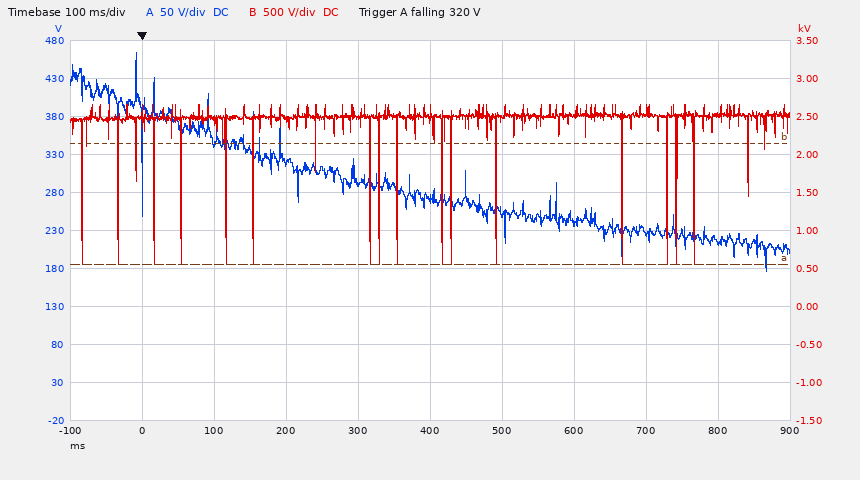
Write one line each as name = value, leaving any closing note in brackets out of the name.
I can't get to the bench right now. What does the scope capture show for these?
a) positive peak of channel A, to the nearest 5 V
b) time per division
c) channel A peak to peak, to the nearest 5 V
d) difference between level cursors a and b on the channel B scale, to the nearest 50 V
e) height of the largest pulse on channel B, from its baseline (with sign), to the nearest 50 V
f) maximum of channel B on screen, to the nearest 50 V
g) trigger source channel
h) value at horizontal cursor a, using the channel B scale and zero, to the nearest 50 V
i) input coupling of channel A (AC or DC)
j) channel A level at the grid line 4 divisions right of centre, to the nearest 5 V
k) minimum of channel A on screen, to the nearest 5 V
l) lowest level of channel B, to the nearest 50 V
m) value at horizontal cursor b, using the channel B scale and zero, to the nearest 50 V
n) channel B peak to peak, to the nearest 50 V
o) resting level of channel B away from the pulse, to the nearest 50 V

positive peak of channel A, to the nearest 5 V = 465 V
time per division = 100 ms
channel A peak to peak, to the nearest 5 V = 290 V
difference between level cursors a and b on the channel B scale, to the nearest 50 V = 1.60 kV
height of the largest pulse on channel B, from its baseline (with sign), to the nearest 50 V = -1.95 kV
maximum of channel B on screen, to the nearest 50 V = 2.65 kV
trigger source channel = channel A
value at horizontal cursor a, using the channel B scale and zero, to the nearest 50 V = 550 V
input coupling of channel A = DC
channel A level at the grid line 4 divisions right of centre, to the nearest 5 V = 215 V
minimum of channel A on screen, to the nearest 5 V = 175 V
lowest level of channel B, to the nearest 50 V = 550 V
value at horizontal cursor b, using the channel B scale and zero, to the nearest 50 V = 2.15 kV
channel B peak to peak, to the nearest 50 V = 2.10 kV
resting level of channel B away from the pulse, to the nearest 50 V = 2.50 kV
